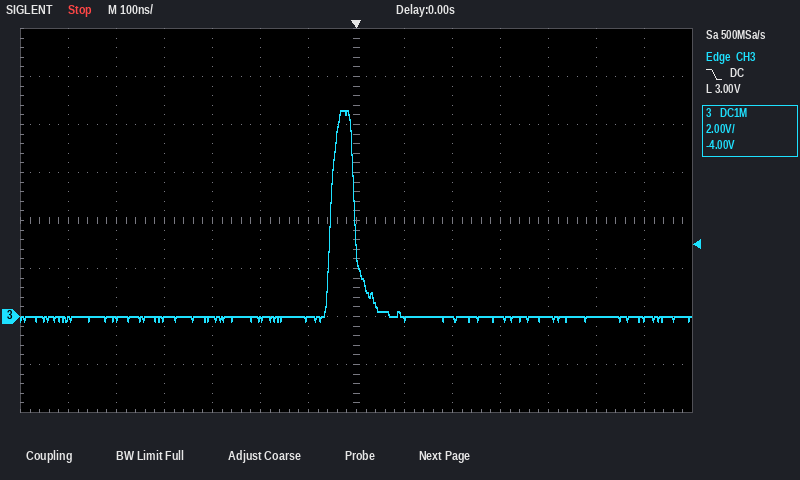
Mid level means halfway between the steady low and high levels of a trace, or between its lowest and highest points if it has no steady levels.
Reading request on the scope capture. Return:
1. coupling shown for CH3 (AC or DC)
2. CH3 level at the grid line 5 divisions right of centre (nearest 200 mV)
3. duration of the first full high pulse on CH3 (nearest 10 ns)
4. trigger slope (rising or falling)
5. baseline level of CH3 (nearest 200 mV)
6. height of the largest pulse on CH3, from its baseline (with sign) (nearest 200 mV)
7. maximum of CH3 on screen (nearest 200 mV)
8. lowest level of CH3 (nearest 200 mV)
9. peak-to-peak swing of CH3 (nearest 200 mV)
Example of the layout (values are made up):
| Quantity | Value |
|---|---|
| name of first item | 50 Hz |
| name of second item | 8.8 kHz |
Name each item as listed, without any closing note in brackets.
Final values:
| Quantity | Value |
|---|---|
| coupling shown for CH3 | DC |
| CH3 level at the grid line 5 divisions right of centre | 0.0 V |
| duration of the first full high pulse on CH3 | 50 ns |
| trigger slope | falling |
| baseline level of CH3 | 0.0 V |
| height of the largest pulse on CH3, from its baseline (with sign) | +8.6 V |
| maximum of CH3 on screen | 8.6 V |
| lowest level of CH3 | -200 mV |
| peak-to-peak swing of CH3 | 8.8 V |
